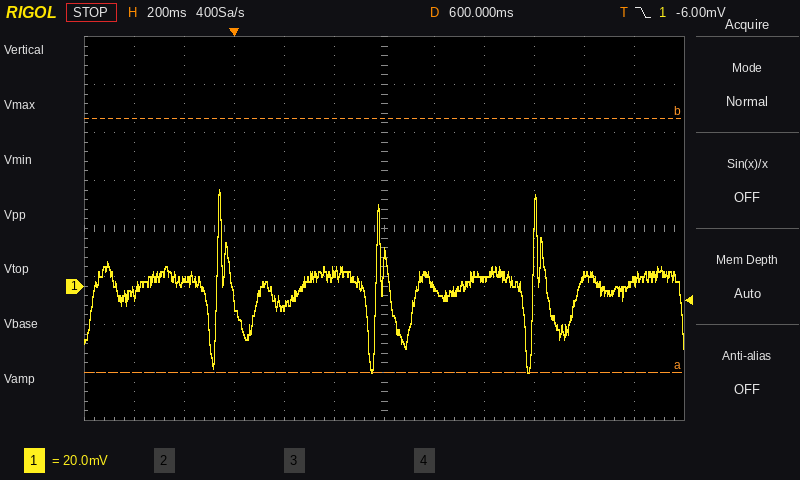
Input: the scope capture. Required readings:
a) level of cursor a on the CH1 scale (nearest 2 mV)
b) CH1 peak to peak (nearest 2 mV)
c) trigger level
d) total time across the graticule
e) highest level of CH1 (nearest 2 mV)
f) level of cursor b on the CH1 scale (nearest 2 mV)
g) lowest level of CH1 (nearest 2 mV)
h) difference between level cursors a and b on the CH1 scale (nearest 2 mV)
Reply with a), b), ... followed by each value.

a) -36 mV
b) 76 mV
c) -6.00 mV
d) 2.4 s
e) 40 mV
f) 70 mV
g) -36 mV
h) 106 mV
